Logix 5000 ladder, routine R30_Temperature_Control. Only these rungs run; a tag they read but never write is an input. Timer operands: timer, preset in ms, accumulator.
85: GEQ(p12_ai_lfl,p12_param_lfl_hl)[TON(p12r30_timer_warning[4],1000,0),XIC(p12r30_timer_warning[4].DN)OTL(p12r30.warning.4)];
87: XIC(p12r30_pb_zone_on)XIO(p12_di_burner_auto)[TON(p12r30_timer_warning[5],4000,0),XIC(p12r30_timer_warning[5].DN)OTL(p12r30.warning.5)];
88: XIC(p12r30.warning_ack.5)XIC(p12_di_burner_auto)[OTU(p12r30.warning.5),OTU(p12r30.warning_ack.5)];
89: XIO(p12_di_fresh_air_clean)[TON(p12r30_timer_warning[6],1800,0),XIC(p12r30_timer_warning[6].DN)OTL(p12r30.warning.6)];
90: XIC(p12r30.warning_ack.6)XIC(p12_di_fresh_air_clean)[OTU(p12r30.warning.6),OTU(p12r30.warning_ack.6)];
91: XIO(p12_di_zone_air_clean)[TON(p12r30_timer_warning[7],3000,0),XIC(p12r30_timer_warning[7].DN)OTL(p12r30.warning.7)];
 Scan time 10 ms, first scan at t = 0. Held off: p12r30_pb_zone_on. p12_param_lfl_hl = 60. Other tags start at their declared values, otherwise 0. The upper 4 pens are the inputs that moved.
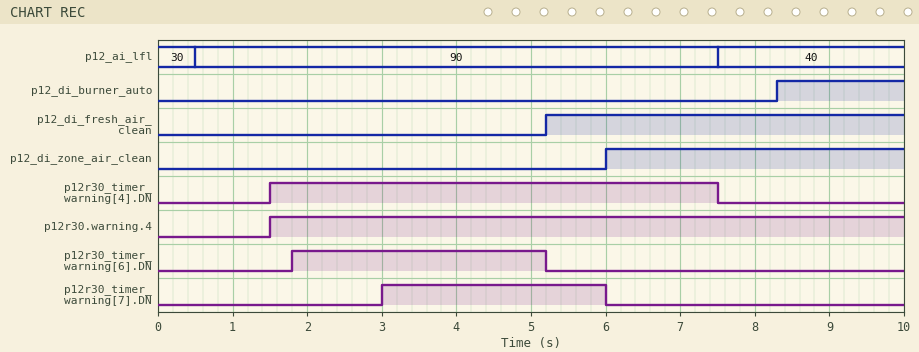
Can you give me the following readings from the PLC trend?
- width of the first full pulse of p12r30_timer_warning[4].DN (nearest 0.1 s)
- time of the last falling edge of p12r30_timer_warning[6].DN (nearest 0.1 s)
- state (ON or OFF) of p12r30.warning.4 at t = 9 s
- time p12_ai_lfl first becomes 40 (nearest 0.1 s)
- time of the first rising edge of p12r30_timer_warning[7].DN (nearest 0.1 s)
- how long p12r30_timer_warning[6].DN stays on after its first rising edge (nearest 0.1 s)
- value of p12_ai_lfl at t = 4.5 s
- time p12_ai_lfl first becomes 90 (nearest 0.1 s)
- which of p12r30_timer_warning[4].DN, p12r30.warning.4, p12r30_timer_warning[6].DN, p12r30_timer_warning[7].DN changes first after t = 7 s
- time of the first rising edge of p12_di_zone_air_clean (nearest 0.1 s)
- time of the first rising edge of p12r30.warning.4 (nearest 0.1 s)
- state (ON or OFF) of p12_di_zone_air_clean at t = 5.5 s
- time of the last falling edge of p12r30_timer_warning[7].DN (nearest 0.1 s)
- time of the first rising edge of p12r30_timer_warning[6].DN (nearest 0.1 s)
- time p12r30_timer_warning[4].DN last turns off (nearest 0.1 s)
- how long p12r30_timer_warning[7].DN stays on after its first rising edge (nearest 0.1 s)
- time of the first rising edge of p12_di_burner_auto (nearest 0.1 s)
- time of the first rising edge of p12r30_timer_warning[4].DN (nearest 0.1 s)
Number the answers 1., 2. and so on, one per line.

1. 6.0 s
2. 5.2 s
3. ON
4. 7.5 s
5. 3.0 s
6. 3.4 s
7. 90
8. 0.5 s
9. p12r30_timer_warning[4].DN
10. 6.0 s
11. 1.5 s
12. OFF
13. 6.0 s
14. 1.8 s
15. 7.5 s
16. 3.0 s
17. 8.3 s
18. 1.5 s
